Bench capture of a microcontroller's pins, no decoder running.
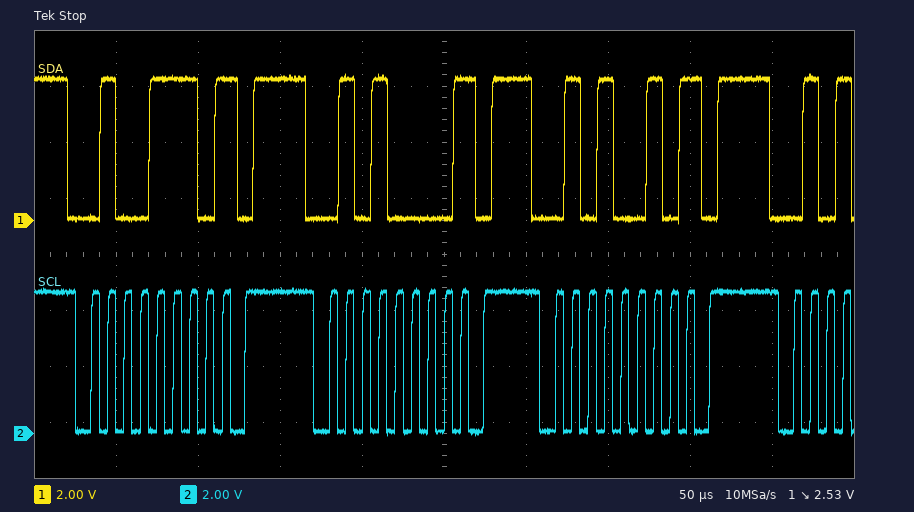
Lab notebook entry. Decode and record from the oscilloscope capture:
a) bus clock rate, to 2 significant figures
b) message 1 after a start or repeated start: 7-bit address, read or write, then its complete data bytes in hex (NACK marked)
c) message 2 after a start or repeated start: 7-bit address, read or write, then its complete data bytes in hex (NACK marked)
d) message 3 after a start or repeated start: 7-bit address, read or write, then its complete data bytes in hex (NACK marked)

100 kHz
0x27 write NACK
0x28 write NACK
0x29 write NACK
